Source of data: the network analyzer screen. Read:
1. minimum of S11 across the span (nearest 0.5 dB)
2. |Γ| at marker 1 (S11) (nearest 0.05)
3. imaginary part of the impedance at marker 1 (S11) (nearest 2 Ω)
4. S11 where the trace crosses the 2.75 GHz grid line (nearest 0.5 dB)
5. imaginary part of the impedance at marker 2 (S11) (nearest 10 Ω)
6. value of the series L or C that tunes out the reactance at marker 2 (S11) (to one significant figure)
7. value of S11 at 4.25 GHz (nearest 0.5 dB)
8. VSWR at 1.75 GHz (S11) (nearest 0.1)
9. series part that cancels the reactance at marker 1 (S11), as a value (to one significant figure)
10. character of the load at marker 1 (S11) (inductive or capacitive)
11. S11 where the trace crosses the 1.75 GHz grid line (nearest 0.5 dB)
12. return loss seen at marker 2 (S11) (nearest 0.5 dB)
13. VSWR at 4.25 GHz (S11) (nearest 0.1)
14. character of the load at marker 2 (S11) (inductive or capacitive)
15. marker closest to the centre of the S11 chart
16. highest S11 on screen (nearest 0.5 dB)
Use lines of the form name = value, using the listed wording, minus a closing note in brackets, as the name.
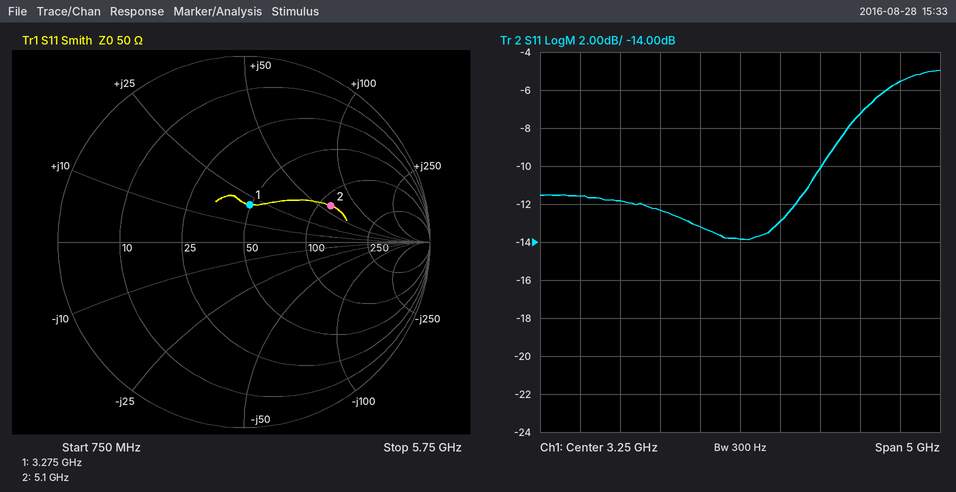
minimum of S11 across the span = -14.0 dB
|Γ| at marker 1 (S11) = 0.20
imaginary part of the impedance at marker 1 (S11) = +20 Ω
S11 where the trace crosses the 2.75 GHz grid line = -13.0 dB
imaginary part of the impedance at marker 2 (S11) = +60 Ω
value of the series L or C that tunes out the reactance at marker 2 (S11) = 500 fF
value of S11 at 4.25 GHz = -10.0 dB
VSWR at 1.75 GHz (S11) = 1.7
series part that cancels the reactance at marker 1 (S11), as a value = 2 pF
character of the load at marker 1 (S11) = inductive
S11 where the trace crosses the 1.75 GHz grid line = -12.0 dB
return loss seen at marker 2 (S11) = 6.0 dB
VSWR at 4.25 GHz (S11) = 1.9
character of the load at marker 2 (S11) = inductive
marker closest to the centre of the S11 chart = marker 1
highest S11 on screen = -5.0 dB
